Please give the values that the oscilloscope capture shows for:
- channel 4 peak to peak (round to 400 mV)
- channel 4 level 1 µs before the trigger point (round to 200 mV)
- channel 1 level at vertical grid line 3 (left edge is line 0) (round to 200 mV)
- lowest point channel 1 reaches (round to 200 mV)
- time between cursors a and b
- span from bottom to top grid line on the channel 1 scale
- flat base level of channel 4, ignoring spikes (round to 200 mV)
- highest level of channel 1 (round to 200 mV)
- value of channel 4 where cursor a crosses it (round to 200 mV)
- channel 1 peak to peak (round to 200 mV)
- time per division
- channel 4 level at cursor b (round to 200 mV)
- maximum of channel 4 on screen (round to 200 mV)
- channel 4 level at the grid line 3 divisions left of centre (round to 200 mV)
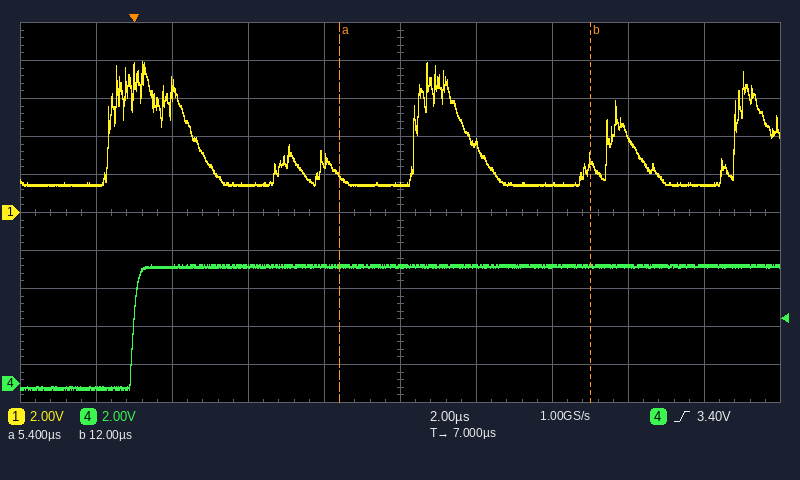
6.4 V
-200 mV
1.4 V
1.4 V
6.6 µs
20 V
-200 mV
8.0 V
6.2 V
6.6 V
2 µs
6.2 V
6.2 V
6.2 V
